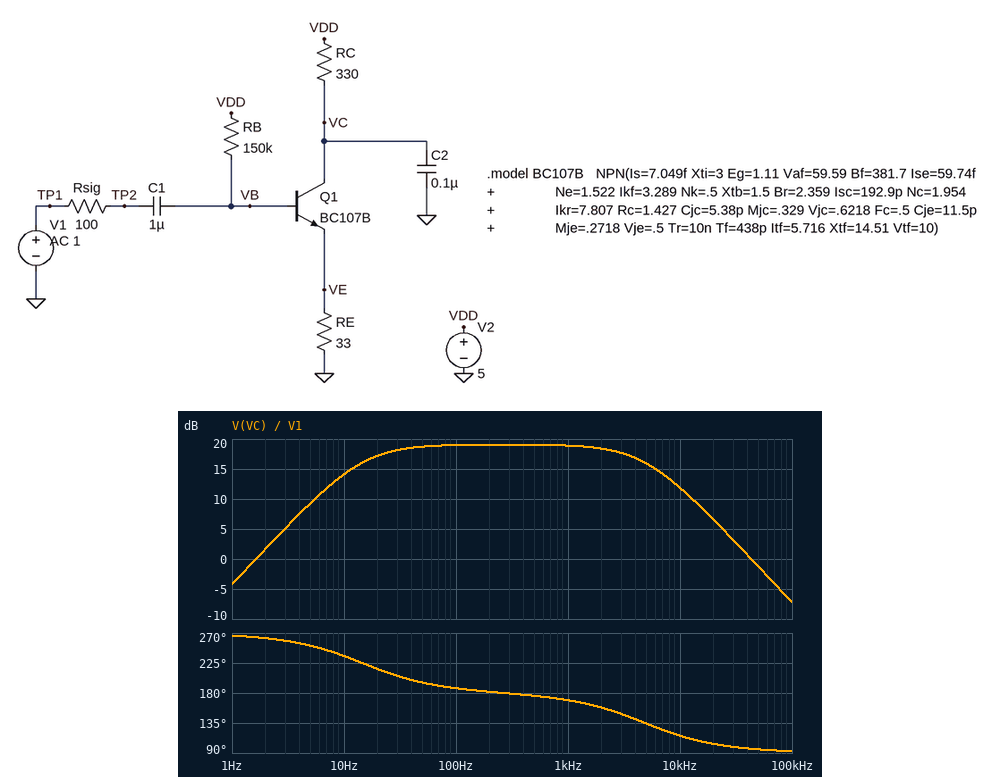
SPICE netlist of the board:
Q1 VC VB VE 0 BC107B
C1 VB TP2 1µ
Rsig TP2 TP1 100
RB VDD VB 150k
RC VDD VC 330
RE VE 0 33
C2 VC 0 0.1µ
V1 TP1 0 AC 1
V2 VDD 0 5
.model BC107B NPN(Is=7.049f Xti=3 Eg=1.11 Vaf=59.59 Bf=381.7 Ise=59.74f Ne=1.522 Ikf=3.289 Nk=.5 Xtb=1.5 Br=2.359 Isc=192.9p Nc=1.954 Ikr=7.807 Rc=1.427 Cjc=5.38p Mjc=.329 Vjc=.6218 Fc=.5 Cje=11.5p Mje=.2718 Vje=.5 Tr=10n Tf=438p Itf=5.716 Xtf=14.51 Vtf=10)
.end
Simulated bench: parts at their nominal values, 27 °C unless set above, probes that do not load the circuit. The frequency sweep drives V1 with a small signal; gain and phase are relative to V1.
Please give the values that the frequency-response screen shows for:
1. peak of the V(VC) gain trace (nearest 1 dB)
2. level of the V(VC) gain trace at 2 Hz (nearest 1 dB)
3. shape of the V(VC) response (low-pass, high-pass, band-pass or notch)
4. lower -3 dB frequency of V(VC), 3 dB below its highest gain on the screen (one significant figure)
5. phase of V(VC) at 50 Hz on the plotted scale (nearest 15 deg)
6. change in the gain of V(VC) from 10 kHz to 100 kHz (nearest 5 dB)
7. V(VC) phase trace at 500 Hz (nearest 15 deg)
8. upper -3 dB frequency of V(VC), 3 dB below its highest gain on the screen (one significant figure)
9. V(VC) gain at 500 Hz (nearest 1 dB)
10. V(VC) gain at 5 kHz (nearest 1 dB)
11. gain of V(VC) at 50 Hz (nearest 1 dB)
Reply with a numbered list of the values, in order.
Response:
1. 19 dB
2. 2 dB
3. band-pass
4. 10 Hz
5. 195 deg
6. -20 dB
7. 180 deg
8. 5 kHz
9. 19 dB
10. 16 dB
11. 19 dB
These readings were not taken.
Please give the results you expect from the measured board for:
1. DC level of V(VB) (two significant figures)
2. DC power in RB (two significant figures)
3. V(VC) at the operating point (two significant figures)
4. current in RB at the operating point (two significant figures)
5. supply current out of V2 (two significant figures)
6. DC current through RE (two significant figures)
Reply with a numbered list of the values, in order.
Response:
1. 1.0 V
2. 110 µW
3. 2.2 V
4. 27 µA
5. 8.4 mA
6. 8.4 mA
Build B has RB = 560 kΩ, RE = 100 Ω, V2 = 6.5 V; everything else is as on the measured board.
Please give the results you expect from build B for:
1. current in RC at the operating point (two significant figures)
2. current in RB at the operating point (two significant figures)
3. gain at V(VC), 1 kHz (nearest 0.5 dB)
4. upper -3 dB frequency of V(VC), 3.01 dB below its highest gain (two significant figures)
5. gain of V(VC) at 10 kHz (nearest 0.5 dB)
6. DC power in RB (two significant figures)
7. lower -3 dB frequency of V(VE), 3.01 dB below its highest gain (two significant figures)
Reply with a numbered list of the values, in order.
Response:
1. 3.0 mA
2. 9.8 µA
3. 9.5 dB
4. 4.8 kHz
5. 2.5 dB
6. 54 µW
7. 4.7 Hz
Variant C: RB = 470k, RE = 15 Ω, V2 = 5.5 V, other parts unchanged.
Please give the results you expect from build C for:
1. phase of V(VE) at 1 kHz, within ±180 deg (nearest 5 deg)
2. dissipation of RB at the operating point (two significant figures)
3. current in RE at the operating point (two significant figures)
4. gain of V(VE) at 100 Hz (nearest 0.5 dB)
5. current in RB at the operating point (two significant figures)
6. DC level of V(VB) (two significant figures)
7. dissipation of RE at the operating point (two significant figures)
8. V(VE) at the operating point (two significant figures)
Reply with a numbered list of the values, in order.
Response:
1. 0 deg
2. 48 µW
3. 3.1 mA
4. -4.0 dB
5. 10 µA
6. 740 mV
7. 140 µW
8. 46 mV
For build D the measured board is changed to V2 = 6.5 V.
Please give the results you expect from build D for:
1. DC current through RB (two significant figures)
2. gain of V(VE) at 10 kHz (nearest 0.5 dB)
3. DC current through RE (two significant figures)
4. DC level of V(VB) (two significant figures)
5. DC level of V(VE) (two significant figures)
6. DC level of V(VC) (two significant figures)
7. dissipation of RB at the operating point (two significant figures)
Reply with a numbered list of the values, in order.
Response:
1. 36 µA
2. -0.5 dB
3. 12 mA
4. 1.1 V
5. 380 mV
6. 2.7 V
7. 190 µW
